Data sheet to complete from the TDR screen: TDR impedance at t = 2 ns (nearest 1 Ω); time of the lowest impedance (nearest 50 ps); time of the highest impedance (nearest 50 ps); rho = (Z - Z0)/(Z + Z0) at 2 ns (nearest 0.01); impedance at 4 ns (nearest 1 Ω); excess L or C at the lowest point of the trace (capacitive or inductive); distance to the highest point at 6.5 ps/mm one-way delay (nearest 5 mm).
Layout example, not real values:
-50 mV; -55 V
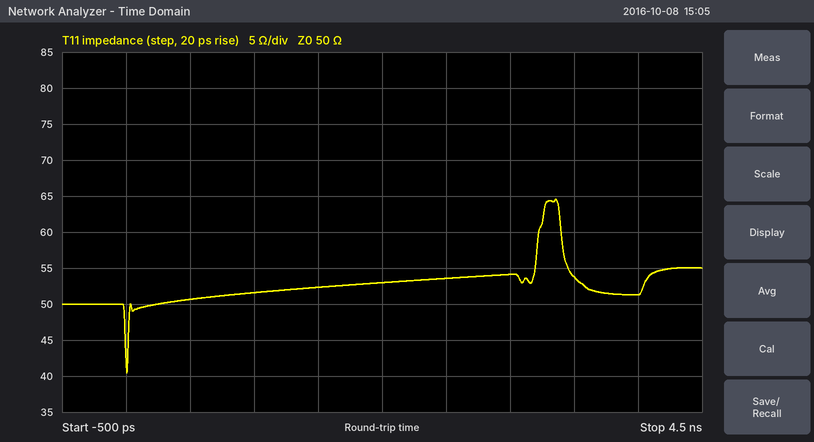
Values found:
53 Ω; 0 ps; 3.35 ns; +0.03; 51 Ω; capacitive; 260 mm
